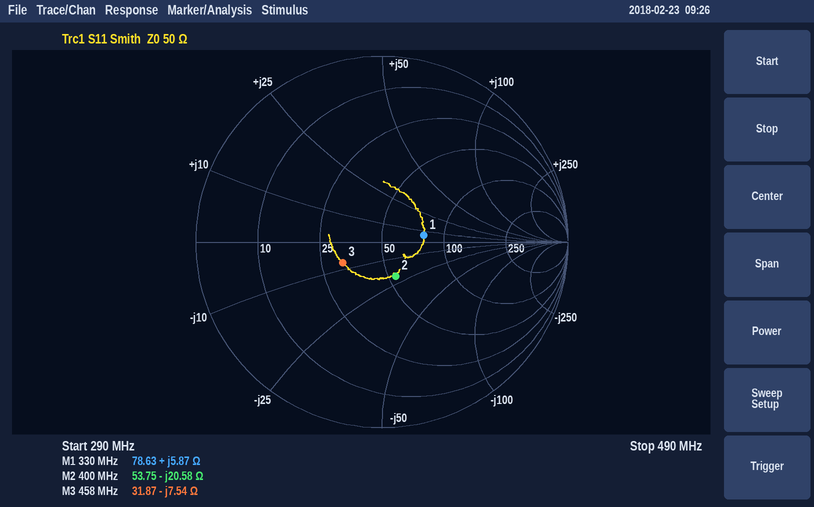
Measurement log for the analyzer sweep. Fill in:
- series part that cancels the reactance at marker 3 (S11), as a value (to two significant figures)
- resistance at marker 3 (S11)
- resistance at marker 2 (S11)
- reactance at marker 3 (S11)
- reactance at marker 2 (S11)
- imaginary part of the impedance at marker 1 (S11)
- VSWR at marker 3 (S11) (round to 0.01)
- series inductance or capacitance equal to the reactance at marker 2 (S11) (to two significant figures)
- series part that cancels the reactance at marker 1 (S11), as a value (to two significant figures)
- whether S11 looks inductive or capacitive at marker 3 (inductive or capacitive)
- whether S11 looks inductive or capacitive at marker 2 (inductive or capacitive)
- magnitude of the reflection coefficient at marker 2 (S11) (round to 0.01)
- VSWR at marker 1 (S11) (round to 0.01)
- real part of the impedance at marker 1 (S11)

2.6 nH
31.87 Ω
53.75 Ω
-7.54 Ω
-20.58 Ω
+5.87 Ω
1.63
19 pF
82 pF
capacitive
capacitive
0.20
1.59
78.63 Ω
